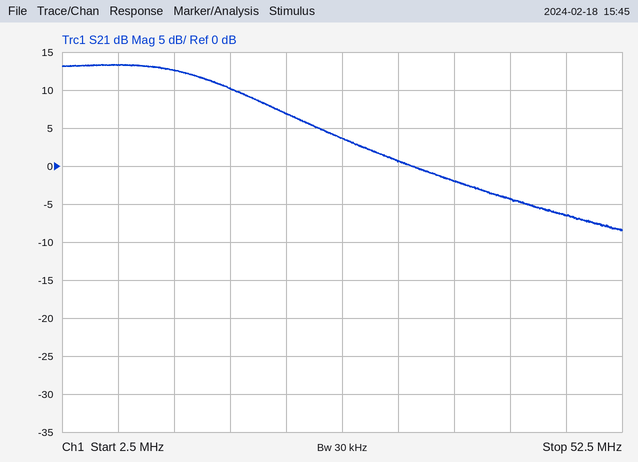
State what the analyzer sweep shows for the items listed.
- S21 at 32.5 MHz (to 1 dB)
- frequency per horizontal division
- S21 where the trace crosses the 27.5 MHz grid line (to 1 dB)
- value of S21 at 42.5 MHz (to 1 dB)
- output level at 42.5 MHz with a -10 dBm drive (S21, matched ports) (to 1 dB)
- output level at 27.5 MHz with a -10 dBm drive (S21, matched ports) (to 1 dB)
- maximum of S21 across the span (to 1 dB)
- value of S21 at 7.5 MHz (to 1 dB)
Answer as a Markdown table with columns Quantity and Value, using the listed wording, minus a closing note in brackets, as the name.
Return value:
| Quantity | Value |
|---|---|
| S21 at 32.5 MHz | 1 dB |
| frequency per horizontal division | 5 MHz |
| S21 where the trace crosses the 27.5 MHz grid line | 4 dB |
| value of S21 at 42.5 MHz | -4 dB |
| output level at 42.5 MHz with a -10 dBm drive (S21, matched ports) | -14 dBm |
| output level at 27.5 MHz with a -10 dBm drive (S21, matched ports) | -6 dBm |
| maximum of S21 across the span | 13 dB |
| value of S21 at 7.5 MHz | 13 dB |
